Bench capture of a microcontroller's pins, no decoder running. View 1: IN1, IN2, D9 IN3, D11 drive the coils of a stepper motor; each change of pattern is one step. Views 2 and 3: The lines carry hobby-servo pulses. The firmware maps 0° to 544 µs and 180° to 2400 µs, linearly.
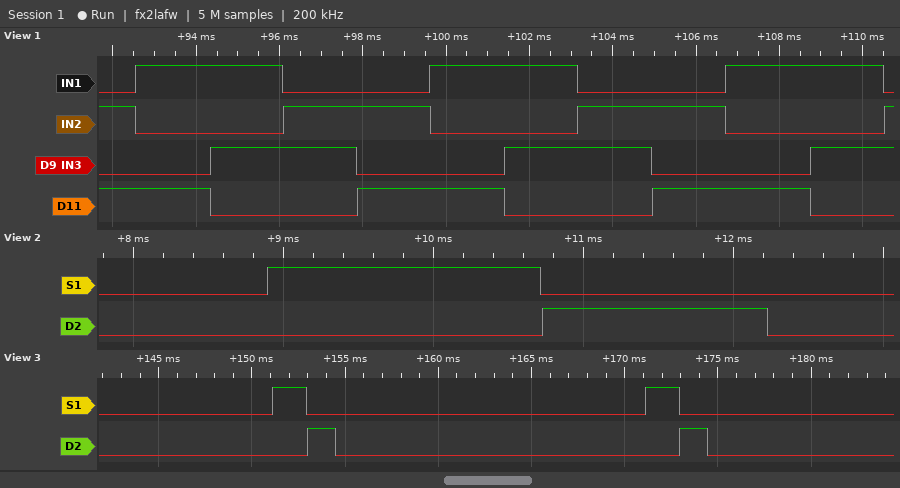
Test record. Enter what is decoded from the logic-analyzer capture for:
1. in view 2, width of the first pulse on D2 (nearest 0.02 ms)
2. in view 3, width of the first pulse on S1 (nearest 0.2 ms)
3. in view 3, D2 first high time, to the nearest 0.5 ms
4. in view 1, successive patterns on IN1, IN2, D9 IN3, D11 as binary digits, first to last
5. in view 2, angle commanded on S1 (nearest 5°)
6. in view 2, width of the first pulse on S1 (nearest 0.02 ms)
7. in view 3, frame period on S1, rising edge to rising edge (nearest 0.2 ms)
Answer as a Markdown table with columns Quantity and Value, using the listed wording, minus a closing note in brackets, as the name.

| Quantity | Value |
|---|---|
| in view 2, width of the first pulse on D2 | 1.50 ms |
| in view 3, width of the first pulse on S1 | 1.8 ms |
| in view 3, D2 first high time, to the nearest 0.5 ms | 1.5 ms |
| in view 1, successive patterns on IN1, IN2, D9 IN3, D11 as binary digits, first to last | 0101 1001 1010 0110 0101 1001 1010 0110 0101 1001 1010 0110 |
| in view 2, angle commanded on S1 | 125° |
| in view 2, width of the first pulse on S1 | 1.82 ms |
| in view 3, frame period on S1, rising edge to rising edge | 20.0 ms |
